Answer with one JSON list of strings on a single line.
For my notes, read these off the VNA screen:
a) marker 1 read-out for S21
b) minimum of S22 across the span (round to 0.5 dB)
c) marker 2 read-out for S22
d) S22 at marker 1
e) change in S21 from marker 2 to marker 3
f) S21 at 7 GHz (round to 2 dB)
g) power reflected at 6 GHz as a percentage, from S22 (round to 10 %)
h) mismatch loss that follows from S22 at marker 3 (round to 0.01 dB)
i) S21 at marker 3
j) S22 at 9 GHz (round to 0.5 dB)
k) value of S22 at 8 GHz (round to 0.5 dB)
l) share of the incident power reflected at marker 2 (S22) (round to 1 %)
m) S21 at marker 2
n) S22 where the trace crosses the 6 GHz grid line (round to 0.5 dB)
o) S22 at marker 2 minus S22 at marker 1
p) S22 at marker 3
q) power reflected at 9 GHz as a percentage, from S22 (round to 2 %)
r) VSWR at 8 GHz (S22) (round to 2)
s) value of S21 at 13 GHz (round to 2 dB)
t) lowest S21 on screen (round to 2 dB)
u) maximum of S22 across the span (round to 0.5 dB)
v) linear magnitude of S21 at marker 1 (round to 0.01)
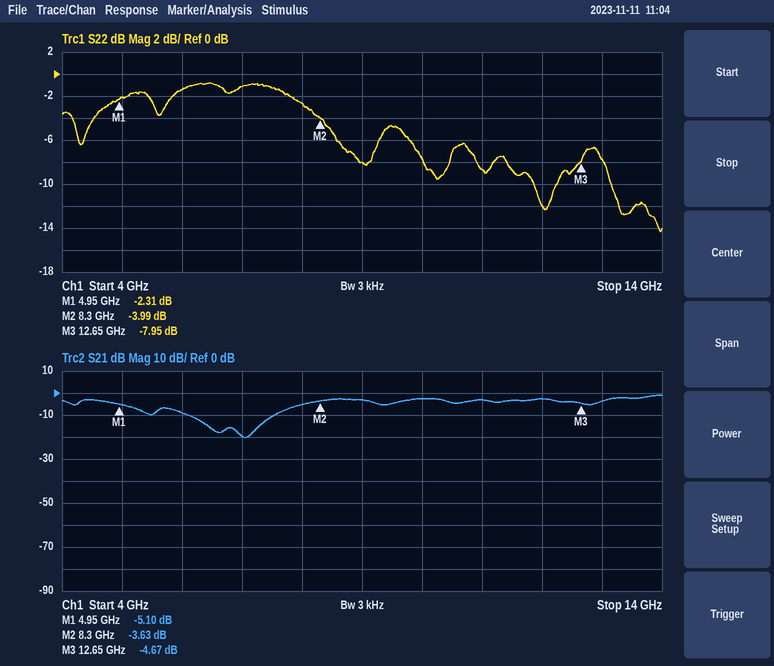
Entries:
["-5.10 dB", "-14.5 dB", "-3.99 dB", "-2.31 dB", "-1.04 dB", "-20 dB", "70 %", "0.76 dB", "-4.67 dB", "-8.0 dB", "-2.5 dB", "40 %", "-3.63 dB", "-1.5 dB", "-1.68 dB", "-7.95 dB", "16 %", "6", "-4 dB", "-20 dB", "-1.0 dB", "0.56"]
